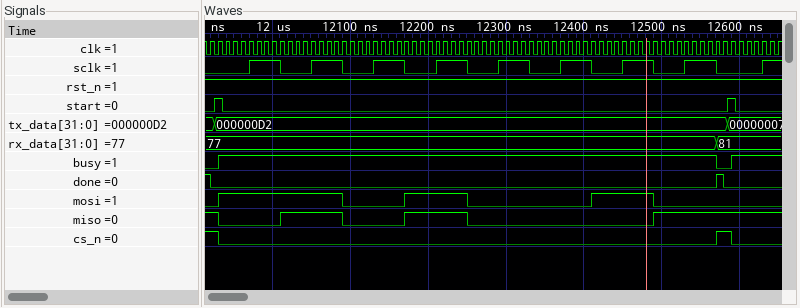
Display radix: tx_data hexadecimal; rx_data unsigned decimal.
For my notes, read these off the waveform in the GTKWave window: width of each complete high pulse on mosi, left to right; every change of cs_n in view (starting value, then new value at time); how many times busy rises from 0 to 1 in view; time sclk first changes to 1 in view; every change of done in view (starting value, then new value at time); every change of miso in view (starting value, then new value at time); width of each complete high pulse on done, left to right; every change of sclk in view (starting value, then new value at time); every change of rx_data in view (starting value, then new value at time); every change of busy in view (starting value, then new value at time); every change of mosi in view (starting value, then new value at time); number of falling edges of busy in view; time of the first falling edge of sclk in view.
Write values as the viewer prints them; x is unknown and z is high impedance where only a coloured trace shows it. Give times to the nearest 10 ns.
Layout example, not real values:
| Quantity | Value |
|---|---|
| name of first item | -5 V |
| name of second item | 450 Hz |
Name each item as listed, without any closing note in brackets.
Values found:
| Quantity | Value |
|---|---|
| width of each complete high pulse on mosi, left to right | 160 ns, 80 ns, 80 ns |
| every change of cs_n in view | 1, 0 at 11930 ns, 1 at 12570 ns, 0 at 12590 ns |
| how many times busy rises from 0 to 1 in view | 2 |
| time sclk first changes to 1 in view | 11970 ns |
| every change of done in view | 1, 0 at 11920 ns, 1 at 12570 ns, 0 at 12580 ns |
| every change of miso in view | 1, 0 at 11930 ns, 1 at 12010 ns, 0 at 12090 ns, 1 at 12170 ns, 0 at 12250 ns, 1 at 12490 ns |
| width of each complete high pulse on done, left to right | 10 ns |
| every change of sclk in view | 0, 1 at 11970 ns, 0 at 12010 ns, 1 at 12050 ns, 0 at 12090 ns, 1 at 12130 ns, 0 at 12170 ns, 1 at 12210 ns, 0 at 12250 ns, 1 at 12290 ns, 0 at 12330 ns, 1 at 12370 ns, 0 at 12410 ns, 1 at 12450 ns, 0 at 12490 ns, 1 at 12530 ns, 0 at 12570 ns, 1 at 12630 ns |
| every change of rx_data in view | 77, 81 at 12570 ns |
| every change of busy in view | 0, 1 at 11930 ns, 0 at 12570 ns, 1 at 12590 ns |
| every change of mosi in view | 0, 1 at 11930 ns, 0 at 12090 ns, 1 at 12170 ns, 0 at 12250 ns, 1 at 12410 ns, 0 at 12490 ns |
| number of falling edges of busy in view | 1 |
| time of the first falling edge of sclk in view | 12010 ns |
